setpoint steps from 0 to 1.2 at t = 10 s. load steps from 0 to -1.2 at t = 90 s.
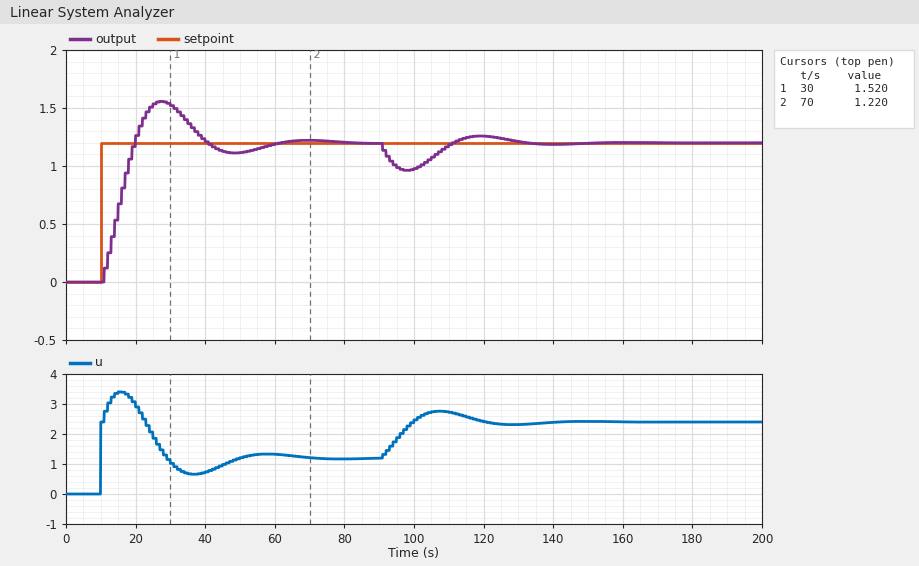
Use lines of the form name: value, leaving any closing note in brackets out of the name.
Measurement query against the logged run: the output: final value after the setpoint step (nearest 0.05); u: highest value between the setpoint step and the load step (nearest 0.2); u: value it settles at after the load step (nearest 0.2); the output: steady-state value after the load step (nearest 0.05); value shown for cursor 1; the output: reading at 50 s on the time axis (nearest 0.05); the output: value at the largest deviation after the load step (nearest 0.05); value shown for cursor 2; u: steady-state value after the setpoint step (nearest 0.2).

the output: final value after the setpoint step: 1.20
u: highest value between the setpoint step and the load step: 3.4
u: value it settles at after the load step: 2.4
the output: steady-state value after the load step: 1.20
value shown for cursor 1: 1.520
the output: reading at 50 s on the time axis: 1.10
the output: value at the largest deviation after the load step: 0.95
value shown for cursor 2: 1.220
u: steady-state value after the setpoint step: 1.2
